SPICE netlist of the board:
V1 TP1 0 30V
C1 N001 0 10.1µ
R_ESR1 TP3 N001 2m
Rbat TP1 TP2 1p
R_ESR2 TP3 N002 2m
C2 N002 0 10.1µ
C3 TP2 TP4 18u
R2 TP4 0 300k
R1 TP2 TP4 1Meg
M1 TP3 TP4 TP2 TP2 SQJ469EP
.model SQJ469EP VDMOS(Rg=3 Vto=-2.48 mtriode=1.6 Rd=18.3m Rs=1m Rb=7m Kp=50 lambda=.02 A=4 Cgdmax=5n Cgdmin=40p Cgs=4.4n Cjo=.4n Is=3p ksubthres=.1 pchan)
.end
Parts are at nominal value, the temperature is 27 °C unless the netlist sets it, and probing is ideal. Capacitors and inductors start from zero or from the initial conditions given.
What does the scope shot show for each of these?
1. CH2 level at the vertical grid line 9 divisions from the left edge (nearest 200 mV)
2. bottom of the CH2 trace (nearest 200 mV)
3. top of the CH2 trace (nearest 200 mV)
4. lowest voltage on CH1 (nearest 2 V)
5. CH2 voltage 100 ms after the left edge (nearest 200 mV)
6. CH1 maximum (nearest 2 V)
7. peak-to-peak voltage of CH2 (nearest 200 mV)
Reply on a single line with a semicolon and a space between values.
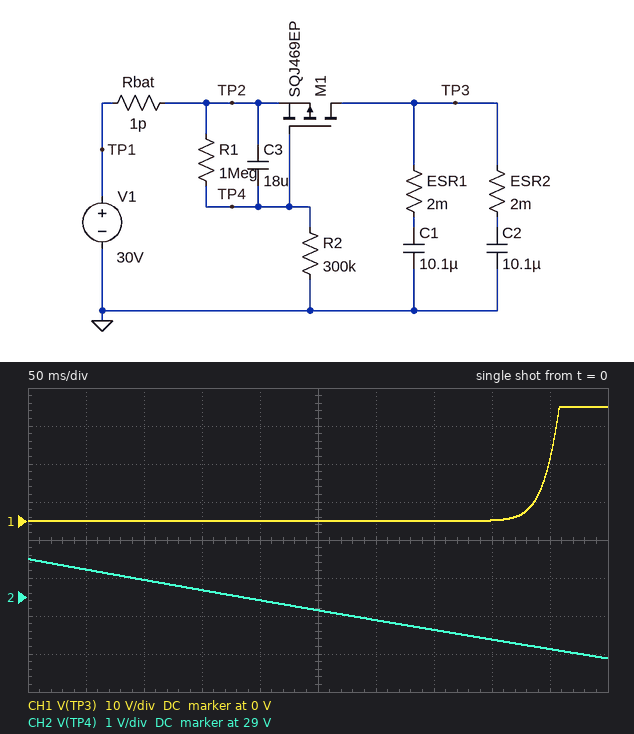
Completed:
27.6 V; 27.4 V; 30.0 V; 0 V; 29.4 V; 30 V; 2.6 V
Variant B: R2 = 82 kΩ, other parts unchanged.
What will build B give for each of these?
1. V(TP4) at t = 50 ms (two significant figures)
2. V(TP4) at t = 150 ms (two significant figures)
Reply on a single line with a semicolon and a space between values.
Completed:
29 V; 27 V
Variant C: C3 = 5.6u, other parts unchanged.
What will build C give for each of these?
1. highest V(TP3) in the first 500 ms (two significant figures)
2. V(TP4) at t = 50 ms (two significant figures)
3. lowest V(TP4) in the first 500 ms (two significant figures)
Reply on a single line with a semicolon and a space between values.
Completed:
30 V; 29 V; 23 V
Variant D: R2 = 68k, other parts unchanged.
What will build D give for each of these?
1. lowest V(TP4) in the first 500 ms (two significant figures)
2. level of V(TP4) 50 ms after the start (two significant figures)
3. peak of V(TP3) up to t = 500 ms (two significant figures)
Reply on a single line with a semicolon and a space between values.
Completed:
20 V; 29 V; 30 V
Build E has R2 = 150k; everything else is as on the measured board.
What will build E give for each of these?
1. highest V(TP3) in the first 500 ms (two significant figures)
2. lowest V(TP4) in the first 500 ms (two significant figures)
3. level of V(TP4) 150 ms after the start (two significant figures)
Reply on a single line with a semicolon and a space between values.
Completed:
30 V; 25 V; 28 V
